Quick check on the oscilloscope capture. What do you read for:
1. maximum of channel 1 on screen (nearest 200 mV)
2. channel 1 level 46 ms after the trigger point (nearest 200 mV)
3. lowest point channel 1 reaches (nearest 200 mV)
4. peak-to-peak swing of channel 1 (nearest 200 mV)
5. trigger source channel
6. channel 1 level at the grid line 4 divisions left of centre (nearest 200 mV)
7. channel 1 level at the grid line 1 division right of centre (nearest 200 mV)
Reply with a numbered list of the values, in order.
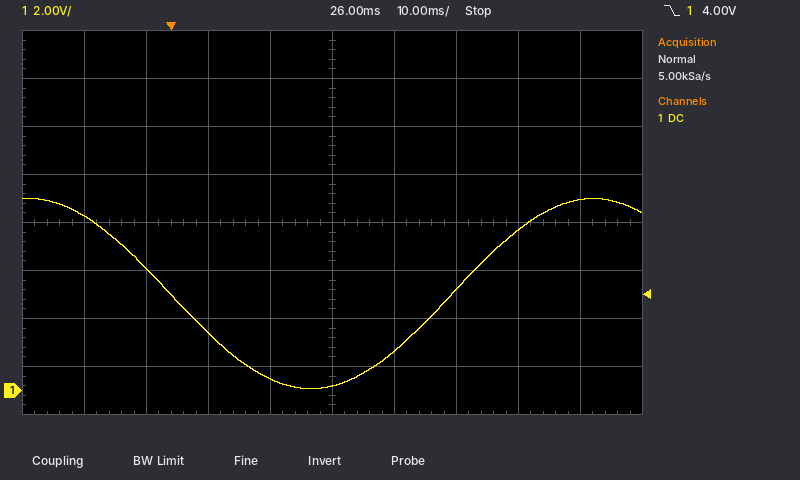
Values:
1. 8.0 V
2. 4.2 V
3. 0.0 V
4. 8.0 V
5. channel 1
6. 7.2 V
7. 1.6 V
